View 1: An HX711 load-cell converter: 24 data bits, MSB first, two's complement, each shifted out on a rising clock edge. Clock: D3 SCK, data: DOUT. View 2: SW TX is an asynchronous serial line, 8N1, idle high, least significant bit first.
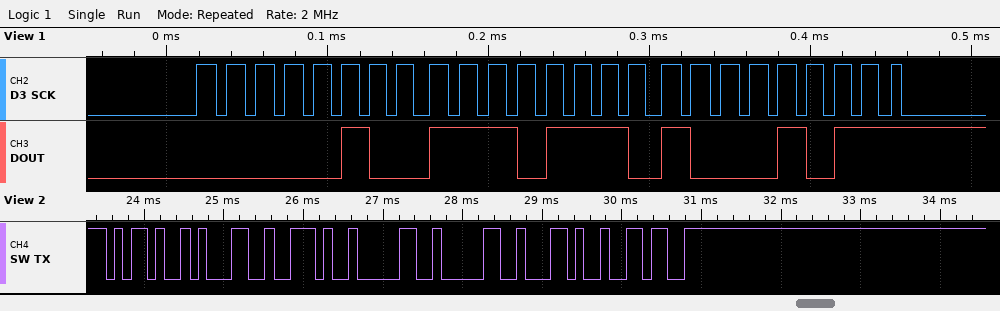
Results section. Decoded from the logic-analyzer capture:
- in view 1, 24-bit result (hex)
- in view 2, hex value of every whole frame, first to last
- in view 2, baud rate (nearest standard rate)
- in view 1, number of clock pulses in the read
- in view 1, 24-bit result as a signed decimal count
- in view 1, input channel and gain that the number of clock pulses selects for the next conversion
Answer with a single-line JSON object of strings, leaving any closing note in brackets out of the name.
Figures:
{"in view 1, 24-bit result": "0x04EE8B", "in view 2, hex value of every whole frame, first to last": "2D 31 2E 30 30 2C 36", "in view 2, baud rate": "9600 baud", "in view 1, number of clock pulses in the read": "25", "in view 1, 24-bit result as a signed decimal count": "323211", "in view 1, input channel and gain that the number of clock pulses selects for the next conversion": "channel A, gain 128"}
